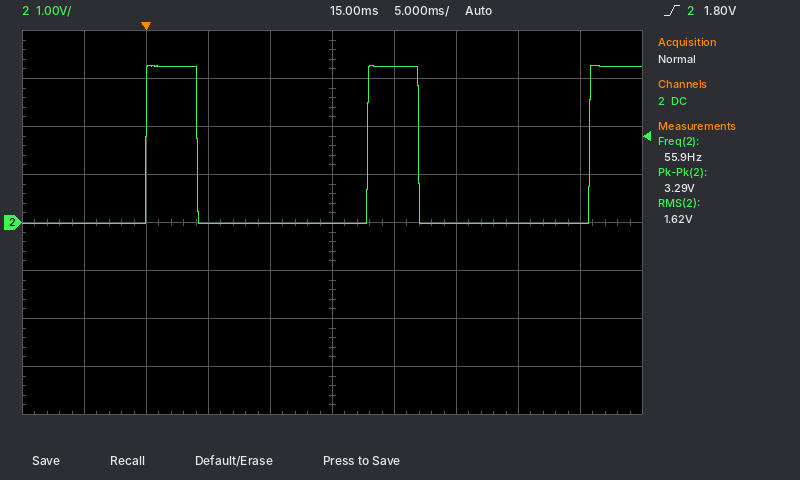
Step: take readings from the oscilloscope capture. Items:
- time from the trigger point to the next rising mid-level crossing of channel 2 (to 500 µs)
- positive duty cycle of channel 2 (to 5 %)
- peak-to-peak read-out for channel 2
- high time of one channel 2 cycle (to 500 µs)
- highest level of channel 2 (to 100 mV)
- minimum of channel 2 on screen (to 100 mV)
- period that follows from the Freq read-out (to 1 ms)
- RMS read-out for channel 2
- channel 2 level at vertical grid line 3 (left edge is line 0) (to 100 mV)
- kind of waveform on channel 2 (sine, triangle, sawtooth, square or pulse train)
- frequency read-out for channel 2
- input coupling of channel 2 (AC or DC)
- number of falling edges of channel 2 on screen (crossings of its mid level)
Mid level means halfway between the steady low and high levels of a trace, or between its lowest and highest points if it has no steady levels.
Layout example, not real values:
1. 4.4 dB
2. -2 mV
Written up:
1. 18.0 ms
2. 25 %
3. 3.29 V
4. 4.0 ms
5. 3.3 V
6. 0.0 V
7. 18 ms
8. 1.62 V
9. 0.0 V
10. pulse train
11. 55.9 Hz
12. DC
13. 2
